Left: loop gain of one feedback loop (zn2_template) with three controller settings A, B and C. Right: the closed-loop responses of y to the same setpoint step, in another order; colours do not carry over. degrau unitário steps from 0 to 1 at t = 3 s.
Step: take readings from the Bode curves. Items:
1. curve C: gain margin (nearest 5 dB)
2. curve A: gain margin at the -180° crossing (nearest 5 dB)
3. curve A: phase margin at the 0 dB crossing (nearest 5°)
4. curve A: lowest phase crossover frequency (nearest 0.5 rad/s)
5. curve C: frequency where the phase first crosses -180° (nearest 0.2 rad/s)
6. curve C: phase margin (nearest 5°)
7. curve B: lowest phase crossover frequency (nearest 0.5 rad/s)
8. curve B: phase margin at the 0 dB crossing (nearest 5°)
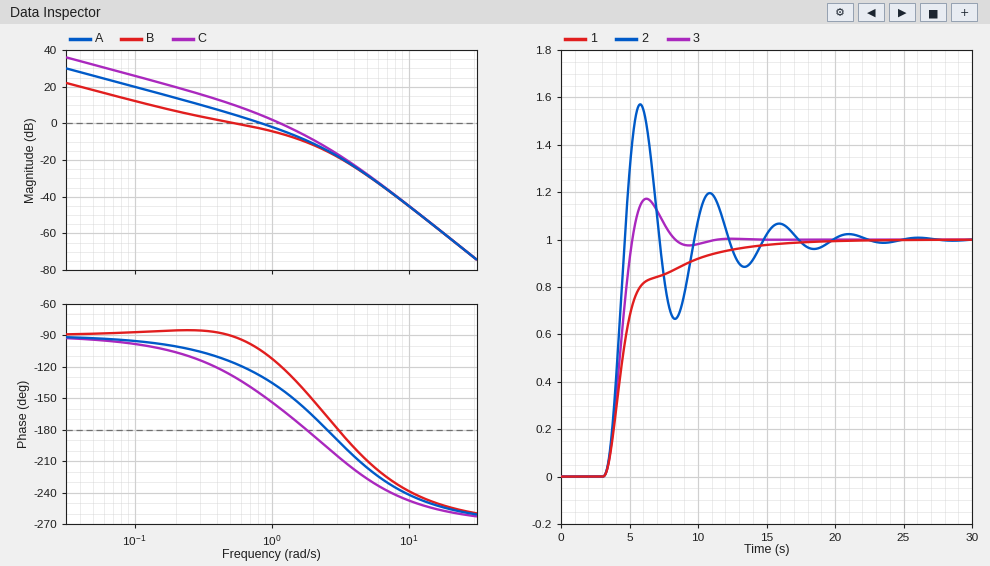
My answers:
5 dB
15 dB
50°
2.5 rad/s
1.8 rad/s
20°
3.0 rad/s
90°
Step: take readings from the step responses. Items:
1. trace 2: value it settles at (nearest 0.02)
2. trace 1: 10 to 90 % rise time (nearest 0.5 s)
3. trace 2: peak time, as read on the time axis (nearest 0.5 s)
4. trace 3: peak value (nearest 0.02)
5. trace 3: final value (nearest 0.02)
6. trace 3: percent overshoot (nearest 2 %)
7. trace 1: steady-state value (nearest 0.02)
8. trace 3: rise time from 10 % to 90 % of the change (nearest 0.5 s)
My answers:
1.00
5.5 s
6.0 s
1.18
1.00
18 %
1.00
1.5 s
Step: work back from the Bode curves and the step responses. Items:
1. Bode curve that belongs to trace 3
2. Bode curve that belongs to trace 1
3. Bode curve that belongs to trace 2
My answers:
A
B
C
